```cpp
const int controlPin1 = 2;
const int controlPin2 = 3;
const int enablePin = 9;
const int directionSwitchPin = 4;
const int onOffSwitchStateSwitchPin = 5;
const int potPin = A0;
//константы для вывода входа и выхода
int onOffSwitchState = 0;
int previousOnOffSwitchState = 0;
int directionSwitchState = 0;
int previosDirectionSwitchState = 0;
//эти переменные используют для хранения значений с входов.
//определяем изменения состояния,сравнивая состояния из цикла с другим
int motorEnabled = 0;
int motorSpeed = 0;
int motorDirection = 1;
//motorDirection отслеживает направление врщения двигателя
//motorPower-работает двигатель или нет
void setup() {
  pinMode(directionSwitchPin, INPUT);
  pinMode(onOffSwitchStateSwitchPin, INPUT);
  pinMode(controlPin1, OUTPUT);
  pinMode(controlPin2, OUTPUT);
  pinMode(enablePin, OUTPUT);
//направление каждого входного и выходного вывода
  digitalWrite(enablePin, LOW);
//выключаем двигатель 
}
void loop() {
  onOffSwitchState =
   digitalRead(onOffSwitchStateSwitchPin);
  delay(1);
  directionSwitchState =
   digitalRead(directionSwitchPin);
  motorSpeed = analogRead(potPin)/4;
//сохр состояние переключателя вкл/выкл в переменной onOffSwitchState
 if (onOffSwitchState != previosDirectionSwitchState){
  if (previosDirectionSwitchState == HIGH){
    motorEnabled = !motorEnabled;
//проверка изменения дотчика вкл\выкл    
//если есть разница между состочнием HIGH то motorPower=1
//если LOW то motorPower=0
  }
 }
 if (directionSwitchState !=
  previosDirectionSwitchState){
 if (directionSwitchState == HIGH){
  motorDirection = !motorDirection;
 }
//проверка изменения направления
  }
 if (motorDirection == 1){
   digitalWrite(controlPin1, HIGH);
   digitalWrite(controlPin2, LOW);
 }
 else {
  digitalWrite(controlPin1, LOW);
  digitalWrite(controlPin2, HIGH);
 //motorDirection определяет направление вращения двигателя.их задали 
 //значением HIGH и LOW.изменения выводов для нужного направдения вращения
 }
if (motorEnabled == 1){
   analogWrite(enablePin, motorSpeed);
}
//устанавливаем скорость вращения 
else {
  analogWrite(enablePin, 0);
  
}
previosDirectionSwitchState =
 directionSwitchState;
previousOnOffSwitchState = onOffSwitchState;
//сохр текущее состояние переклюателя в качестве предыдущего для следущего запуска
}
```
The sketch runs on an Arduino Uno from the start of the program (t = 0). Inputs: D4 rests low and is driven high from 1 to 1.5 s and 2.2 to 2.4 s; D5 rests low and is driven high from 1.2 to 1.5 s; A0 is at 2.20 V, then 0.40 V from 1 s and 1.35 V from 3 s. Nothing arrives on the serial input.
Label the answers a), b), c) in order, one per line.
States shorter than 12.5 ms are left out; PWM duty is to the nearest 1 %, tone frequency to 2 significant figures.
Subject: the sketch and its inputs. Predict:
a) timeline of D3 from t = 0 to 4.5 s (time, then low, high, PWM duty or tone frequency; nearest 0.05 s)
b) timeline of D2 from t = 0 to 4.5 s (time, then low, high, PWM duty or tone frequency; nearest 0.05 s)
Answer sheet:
a) 0 s low; 1 s high; 2.2 s low
b) 0 s high; 1 s low; 2.2 s high
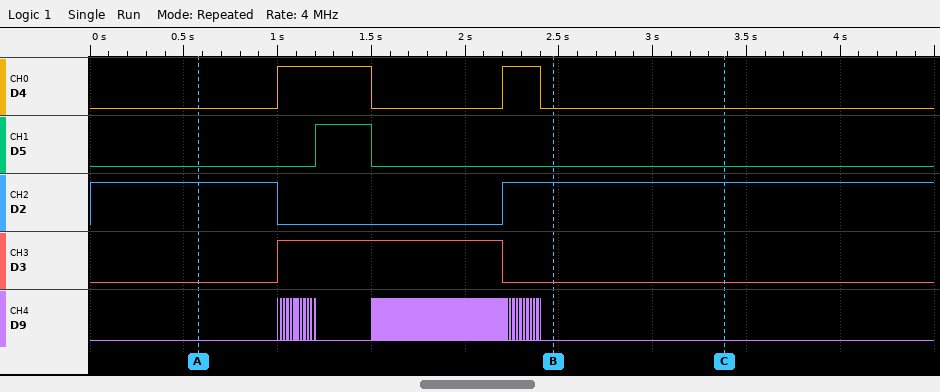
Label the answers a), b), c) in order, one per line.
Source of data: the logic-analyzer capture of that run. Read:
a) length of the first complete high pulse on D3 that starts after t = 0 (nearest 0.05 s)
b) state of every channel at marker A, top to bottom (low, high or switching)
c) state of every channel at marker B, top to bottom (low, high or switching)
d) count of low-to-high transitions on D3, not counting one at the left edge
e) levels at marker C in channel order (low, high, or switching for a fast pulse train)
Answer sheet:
a) 1.20 s
b) D4 low, D5 low, D2 high, D3 low, D9 low
c) D4 low, D5 low, D2 high, D3 low, D9 low
d) 1
e) D4 low, D5 low, D2 high, D3 low, D9 low
